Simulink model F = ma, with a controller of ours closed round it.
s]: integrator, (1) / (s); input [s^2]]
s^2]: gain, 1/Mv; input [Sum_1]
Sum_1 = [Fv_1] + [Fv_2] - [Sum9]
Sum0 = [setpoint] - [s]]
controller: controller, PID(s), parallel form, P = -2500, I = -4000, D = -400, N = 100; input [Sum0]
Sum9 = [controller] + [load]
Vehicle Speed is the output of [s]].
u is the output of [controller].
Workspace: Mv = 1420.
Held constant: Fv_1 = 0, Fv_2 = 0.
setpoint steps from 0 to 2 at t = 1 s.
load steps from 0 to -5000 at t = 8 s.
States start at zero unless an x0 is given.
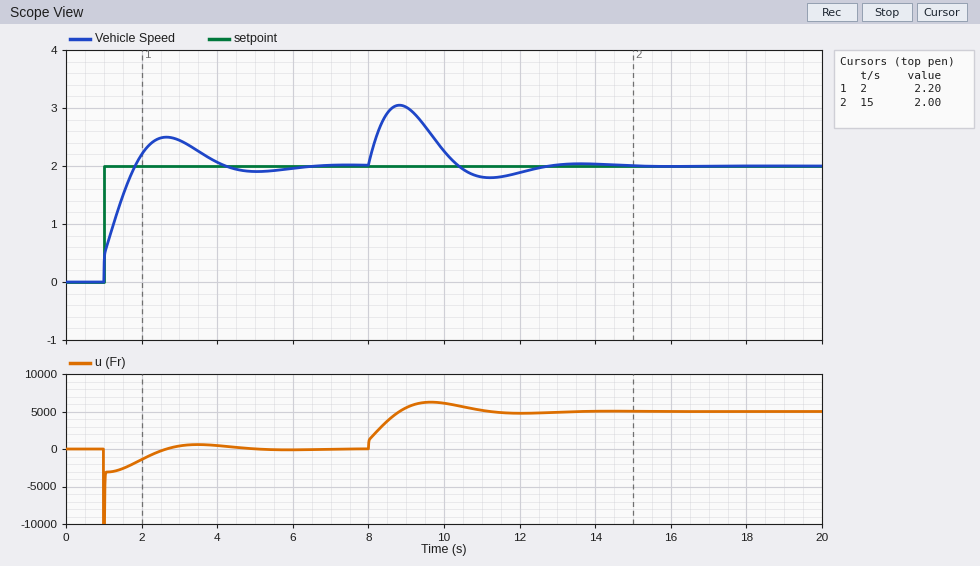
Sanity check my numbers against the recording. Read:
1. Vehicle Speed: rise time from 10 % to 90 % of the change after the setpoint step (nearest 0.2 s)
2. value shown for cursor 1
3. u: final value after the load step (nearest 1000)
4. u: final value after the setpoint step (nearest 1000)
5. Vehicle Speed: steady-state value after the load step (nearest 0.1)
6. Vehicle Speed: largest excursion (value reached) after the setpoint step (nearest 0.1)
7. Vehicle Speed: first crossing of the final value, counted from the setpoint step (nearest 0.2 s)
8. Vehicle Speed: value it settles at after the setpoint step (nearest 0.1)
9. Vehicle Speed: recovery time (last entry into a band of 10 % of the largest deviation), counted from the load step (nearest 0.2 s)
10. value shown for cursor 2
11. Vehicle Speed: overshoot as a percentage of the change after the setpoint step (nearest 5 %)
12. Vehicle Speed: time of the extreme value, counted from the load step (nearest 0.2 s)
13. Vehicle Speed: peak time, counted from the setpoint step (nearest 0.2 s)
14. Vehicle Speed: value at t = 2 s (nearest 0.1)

0.6 s
2.20
5000
0
2.0
2.5
0.8 s
2.0
4.0 s
2.00
25 %
0.8 s
1.6 s
2.2
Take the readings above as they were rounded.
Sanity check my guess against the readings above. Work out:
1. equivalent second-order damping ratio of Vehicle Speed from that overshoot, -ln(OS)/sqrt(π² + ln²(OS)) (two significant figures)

0.40
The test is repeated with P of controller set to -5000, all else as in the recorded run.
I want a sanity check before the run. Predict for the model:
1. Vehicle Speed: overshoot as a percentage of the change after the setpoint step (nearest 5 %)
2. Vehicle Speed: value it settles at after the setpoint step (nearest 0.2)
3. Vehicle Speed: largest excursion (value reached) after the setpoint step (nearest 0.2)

10 %
2.0
2.2
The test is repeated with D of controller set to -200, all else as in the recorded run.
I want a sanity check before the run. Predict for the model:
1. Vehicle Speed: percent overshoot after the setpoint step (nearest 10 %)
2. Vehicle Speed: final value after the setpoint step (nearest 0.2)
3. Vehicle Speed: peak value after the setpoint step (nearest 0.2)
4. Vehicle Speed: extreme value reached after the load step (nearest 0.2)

30 %
2.0
2.6
3.0
